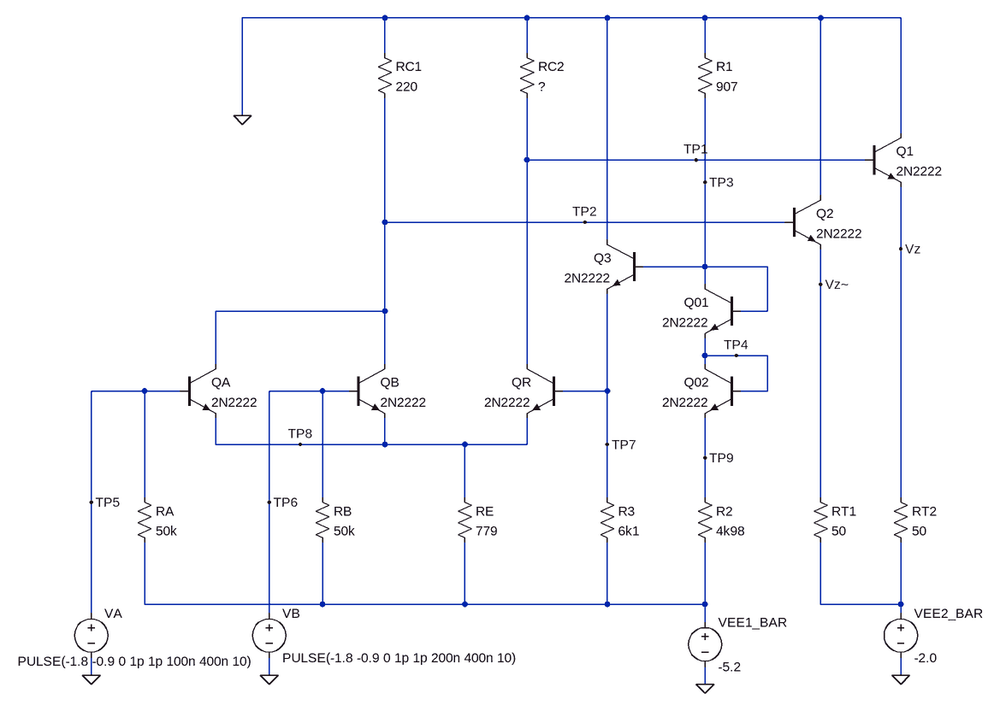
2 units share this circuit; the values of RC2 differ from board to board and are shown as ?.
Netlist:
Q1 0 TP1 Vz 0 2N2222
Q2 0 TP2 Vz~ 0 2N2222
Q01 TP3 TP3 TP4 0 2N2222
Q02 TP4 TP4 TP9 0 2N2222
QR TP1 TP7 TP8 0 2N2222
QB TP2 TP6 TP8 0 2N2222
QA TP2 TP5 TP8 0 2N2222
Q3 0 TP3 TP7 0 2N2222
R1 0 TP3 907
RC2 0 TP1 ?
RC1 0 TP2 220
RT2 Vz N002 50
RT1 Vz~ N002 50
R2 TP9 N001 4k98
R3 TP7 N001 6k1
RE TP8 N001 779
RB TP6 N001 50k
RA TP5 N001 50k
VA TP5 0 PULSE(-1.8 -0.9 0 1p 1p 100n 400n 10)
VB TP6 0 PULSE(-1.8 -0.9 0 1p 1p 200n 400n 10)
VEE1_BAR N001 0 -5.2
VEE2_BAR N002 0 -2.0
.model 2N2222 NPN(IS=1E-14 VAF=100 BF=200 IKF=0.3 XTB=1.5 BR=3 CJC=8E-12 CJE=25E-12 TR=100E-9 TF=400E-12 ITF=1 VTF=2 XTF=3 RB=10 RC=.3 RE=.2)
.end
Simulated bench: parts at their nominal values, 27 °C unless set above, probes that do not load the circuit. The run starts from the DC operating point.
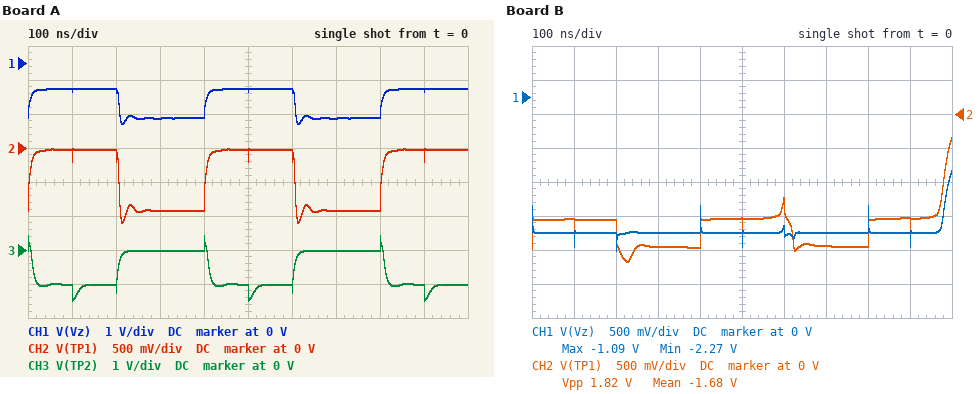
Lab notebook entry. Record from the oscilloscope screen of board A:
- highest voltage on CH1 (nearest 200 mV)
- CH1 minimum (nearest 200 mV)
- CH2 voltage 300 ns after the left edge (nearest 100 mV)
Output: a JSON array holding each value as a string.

["-800 mV", "-1.8 V", "-900 mV"]
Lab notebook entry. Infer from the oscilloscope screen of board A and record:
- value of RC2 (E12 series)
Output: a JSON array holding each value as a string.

["220 Ω"]
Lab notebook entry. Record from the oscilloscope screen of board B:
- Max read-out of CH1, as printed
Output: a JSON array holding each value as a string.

["-1.09 V"]
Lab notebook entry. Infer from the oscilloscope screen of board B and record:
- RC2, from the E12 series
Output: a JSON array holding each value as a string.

["680 Ω"]
